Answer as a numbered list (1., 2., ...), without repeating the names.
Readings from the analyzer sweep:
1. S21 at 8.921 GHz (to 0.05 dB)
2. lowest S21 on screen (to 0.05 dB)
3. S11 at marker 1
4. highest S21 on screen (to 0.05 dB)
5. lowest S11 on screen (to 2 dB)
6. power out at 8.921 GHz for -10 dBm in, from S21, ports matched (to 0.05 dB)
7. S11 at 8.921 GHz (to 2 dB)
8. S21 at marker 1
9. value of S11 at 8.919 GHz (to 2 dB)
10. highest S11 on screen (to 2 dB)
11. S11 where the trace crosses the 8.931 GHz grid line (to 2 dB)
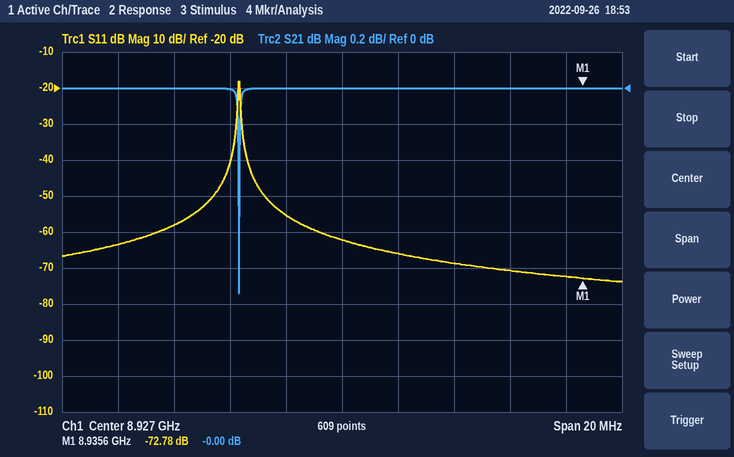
1. 0.00 dB
2. -1.15 dB
3. -72.78 dB
4. 0.00 dB
5. -74 dB
6. -10.00 dBm
7. -58 dB
8. -0.00 dB
9. -64 dB
10. -18 dB
11. -68 dB
